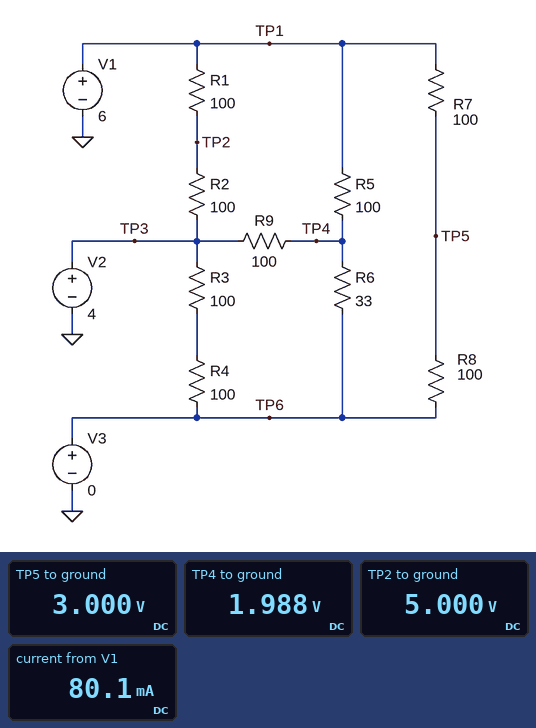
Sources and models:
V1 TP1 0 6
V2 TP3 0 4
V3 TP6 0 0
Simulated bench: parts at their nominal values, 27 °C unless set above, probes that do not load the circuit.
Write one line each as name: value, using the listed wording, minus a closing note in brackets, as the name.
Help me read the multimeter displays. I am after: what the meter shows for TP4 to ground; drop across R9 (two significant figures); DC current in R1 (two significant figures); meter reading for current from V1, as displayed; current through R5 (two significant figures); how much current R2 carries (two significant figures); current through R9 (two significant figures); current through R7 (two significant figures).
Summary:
what the meter shows for TP4 to ground: 1.988 V
drop across R9: 2.0 V
DC current in R1: 10 mA
meter reading for current from V1, as displayed: 80.1 mA
current through R5: 40 mA
how much current R2 carries: 10 mA
current through R9: 20 mA
current through R7: 30 mA
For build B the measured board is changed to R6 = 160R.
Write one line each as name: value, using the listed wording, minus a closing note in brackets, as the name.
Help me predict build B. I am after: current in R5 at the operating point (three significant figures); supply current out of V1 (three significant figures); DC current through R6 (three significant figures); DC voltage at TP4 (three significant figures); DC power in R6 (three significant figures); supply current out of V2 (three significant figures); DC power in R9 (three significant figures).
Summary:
current in R5 at the operating point: 21.9 mA
supply current out of V1: 61.9 mA
DC current through R6: 23.8 mA
DC voltage at TP4: 3.81 V
DC power in R6: 90.7 mW
supply current out of V2: 11.9 mA
DC power in R9: 363 µW
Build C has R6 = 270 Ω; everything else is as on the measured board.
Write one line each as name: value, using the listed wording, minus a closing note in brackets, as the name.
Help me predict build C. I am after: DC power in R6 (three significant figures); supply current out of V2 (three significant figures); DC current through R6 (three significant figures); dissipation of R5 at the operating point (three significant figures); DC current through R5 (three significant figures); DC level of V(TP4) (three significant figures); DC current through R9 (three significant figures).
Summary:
DC power in R6: 65.9 mW
supply current out of V2: 7.81 mA
DC current through R6: 15.6 mA
dissipation of R5 at the operating point: 31.7 mW
DC current through R5: 17.8 mA
DC level of V(TP4): 4.22 V
DC current through R9: 2.19 mA
